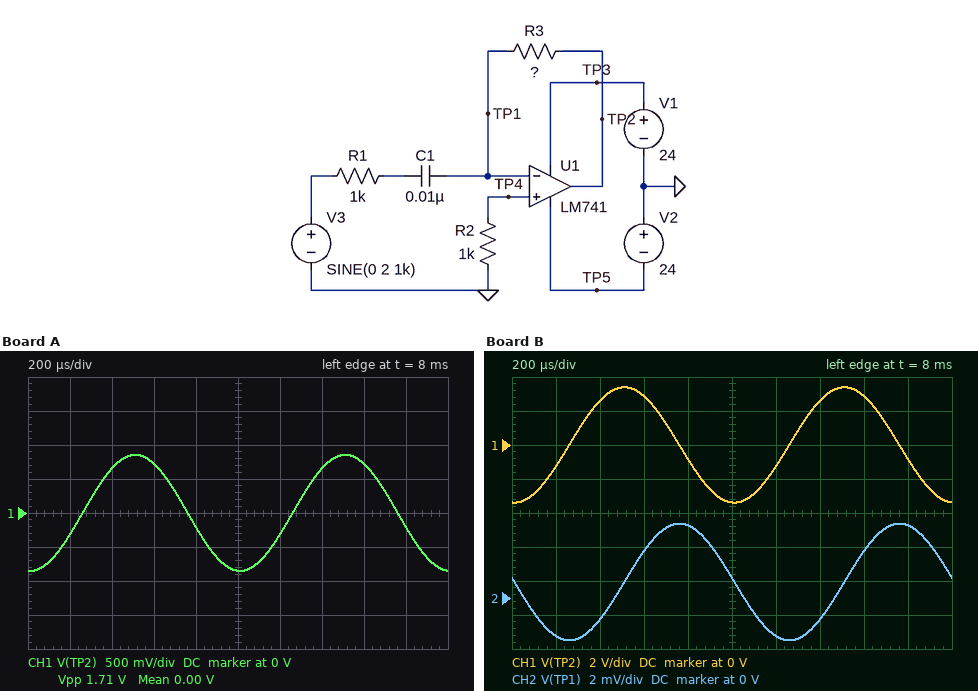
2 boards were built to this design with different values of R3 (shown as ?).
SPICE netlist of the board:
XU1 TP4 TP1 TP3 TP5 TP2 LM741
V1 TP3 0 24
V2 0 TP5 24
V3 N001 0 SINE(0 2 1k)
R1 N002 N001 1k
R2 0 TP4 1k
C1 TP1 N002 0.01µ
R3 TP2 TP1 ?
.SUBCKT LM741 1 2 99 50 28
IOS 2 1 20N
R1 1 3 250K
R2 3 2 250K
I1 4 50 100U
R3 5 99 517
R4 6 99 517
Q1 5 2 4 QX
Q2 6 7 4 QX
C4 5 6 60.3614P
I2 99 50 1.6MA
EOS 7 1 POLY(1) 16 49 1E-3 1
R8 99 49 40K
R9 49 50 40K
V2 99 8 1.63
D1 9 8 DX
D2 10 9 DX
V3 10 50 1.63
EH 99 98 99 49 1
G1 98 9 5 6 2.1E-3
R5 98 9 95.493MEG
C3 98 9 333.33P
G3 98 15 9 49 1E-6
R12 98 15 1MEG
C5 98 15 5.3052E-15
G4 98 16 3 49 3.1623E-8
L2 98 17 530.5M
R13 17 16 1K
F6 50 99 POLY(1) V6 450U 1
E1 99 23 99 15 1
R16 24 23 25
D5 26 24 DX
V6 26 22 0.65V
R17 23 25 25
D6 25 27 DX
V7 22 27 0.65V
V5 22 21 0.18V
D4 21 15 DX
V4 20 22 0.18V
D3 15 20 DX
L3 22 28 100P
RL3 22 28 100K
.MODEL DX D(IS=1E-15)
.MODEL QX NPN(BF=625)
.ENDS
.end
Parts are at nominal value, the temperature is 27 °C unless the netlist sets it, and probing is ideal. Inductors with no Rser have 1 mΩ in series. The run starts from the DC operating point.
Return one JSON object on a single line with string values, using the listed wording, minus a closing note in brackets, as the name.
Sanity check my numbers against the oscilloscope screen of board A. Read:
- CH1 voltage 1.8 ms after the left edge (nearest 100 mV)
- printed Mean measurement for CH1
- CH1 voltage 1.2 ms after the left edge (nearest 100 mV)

{"CH1 voltage 1.8 ms after the left edge": "-200 mV", "printed Mean measurement for CH1": "0.00 V", "CH1 voltage 1.2 ms after the left edge": "-300 mV"}
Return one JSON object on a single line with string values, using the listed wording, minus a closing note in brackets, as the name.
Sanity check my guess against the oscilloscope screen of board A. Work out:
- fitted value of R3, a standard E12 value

{"fitted value of R3, a standard E12 value": "6.8 kΩ"}
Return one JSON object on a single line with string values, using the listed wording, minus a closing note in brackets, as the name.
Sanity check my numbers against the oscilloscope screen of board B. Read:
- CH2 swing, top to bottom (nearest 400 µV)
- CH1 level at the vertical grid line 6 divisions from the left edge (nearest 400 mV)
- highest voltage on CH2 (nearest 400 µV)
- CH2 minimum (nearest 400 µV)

{"CH2 swing, top to bottom": "6.8 mV", "CH1 level at the vertical grid line 6 divisions from the left edge": "-1.2 V", "highest voltage on CH2": "4.4 mV", "CH2 minimum": "-2.4 mV"}
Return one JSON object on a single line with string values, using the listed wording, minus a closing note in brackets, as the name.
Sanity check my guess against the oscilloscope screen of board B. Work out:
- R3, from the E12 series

{"R3, from the E12 series": "27 kΩ"}
